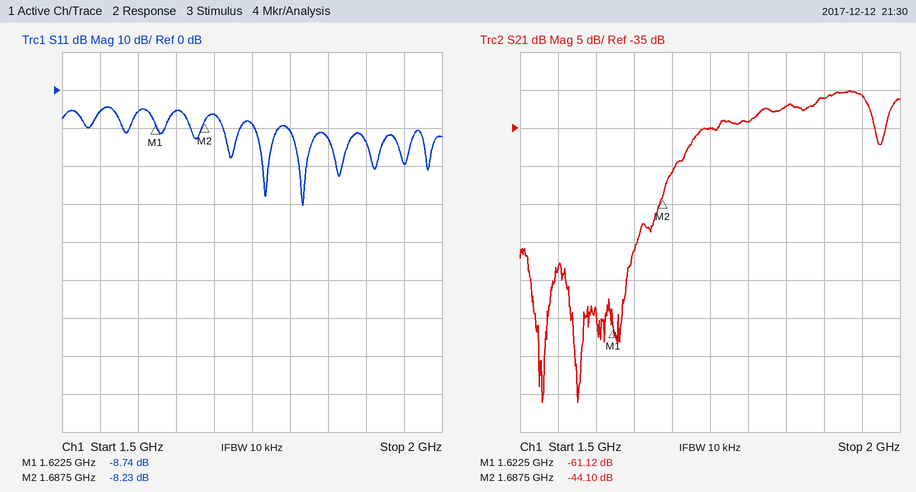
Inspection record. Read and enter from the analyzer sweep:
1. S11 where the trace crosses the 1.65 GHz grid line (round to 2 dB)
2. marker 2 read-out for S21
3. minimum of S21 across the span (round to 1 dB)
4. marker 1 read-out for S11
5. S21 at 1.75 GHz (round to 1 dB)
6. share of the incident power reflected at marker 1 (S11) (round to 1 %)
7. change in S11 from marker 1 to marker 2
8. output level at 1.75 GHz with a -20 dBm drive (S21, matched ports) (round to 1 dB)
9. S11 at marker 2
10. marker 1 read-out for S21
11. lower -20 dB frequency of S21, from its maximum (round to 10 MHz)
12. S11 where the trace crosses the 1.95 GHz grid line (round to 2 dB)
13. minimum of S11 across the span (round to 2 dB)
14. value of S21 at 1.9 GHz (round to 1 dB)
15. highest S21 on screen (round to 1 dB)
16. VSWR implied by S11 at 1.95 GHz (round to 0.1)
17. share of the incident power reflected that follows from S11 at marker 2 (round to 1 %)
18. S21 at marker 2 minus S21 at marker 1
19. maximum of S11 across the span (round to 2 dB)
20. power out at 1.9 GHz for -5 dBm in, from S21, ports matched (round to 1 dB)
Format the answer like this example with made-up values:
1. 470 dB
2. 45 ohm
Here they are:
1. -6 dB
2. -44.10 dB
3. -71 dB
4. -8.74 dB
5. -35 dB
6. 13 %
7. 0.51 dB
8. -55 dBm
9. -8.23 dB
10. -61.12 dB
11. 1.65 GHz
12. -20 dB
13. -30 dB
14. -31 dB
15. -30 dB
16. 1.2
17. 15 %
18. 17.02 dB
19. -4 dB
20. -36 dBm
